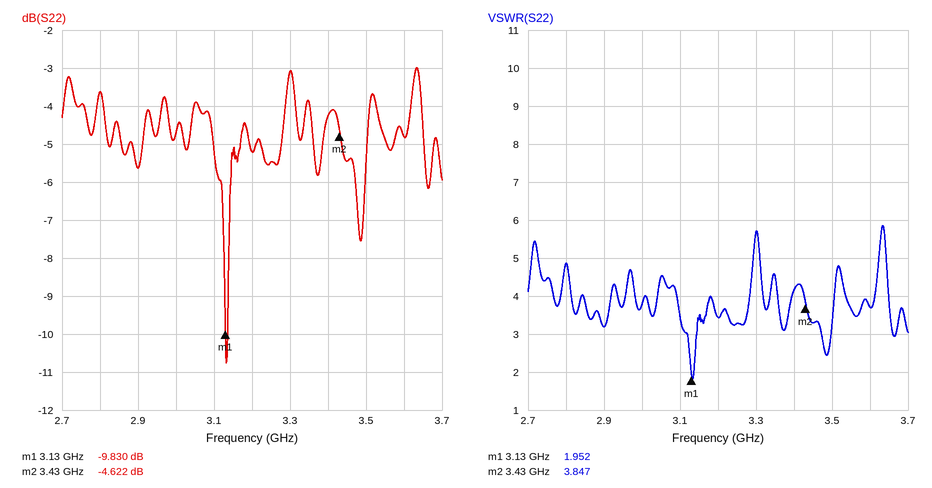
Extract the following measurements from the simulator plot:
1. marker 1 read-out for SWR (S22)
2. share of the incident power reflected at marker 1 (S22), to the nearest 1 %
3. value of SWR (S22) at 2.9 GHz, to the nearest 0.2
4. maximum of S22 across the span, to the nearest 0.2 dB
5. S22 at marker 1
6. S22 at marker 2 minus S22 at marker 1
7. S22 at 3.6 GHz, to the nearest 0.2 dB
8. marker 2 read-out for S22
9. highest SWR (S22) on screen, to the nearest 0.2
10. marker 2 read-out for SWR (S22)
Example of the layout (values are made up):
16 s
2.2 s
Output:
1.952
10 %
3.2
-3.0 dB
-9.830 dB
5.208 dB
-4.8 dB
-4.622 dB
5.8
3.847
